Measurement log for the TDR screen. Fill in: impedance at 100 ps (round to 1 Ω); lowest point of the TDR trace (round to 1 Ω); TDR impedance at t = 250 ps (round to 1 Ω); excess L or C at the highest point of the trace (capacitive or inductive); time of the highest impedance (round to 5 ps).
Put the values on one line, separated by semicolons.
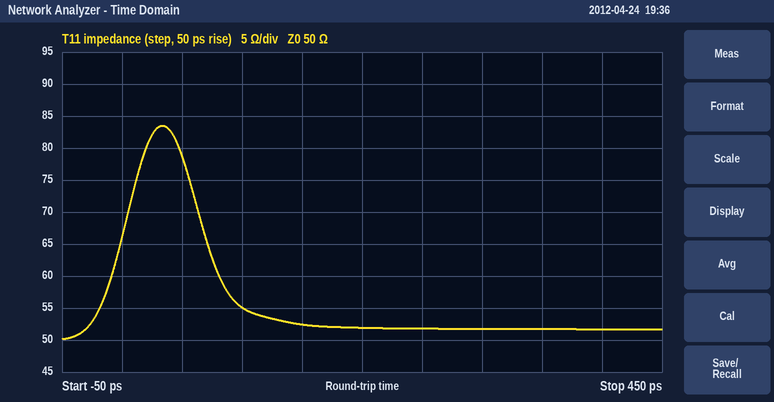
55 Ω; 50 Ω; 52 Ω; inductive; 35 ps
